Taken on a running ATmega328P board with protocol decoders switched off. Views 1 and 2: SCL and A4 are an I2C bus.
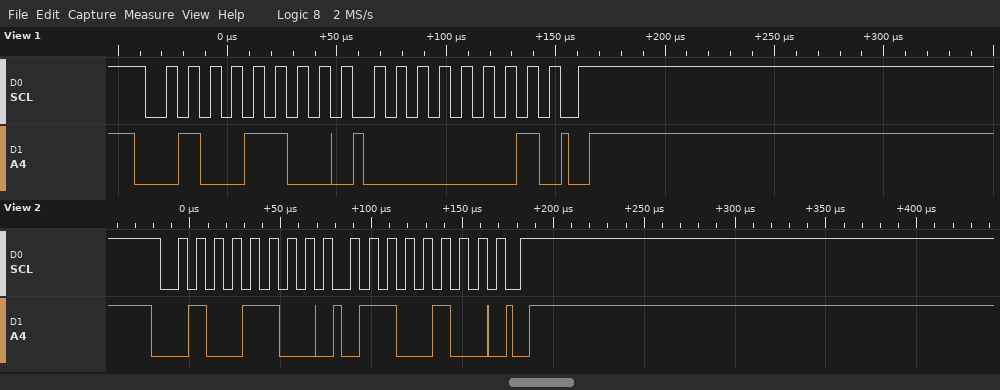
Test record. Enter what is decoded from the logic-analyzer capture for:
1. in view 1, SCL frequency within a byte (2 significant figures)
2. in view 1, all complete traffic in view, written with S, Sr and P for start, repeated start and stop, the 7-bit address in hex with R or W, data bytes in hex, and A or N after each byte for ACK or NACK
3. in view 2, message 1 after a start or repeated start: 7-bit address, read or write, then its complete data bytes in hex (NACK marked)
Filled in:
100 kHz
S 26W A 01 A P
0x26 write: 64
